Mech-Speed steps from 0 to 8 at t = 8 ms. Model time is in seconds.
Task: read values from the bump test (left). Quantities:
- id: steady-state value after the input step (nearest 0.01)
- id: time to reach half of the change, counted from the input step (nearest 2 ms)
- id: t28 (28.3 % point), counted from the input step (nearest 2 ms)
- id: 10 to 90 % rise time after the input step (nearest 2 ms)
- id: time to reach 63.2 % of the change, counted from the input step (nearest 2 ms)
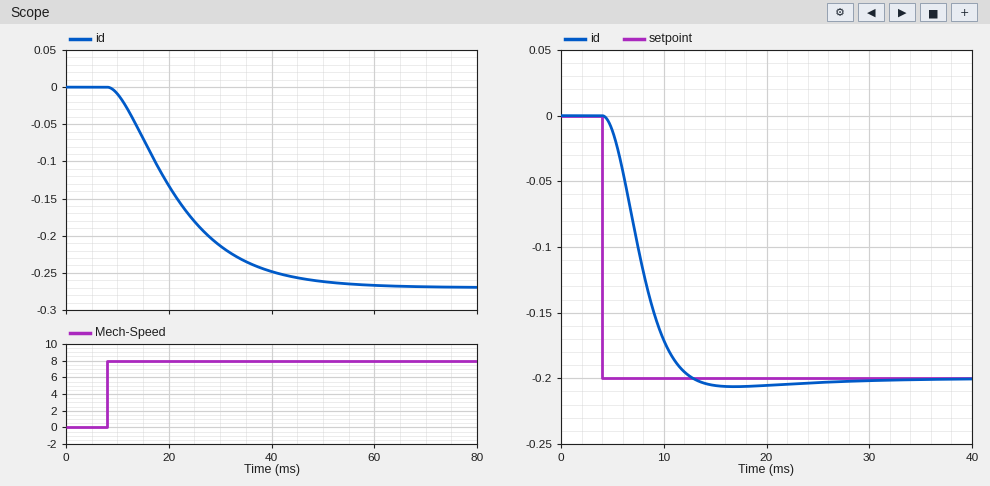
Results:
-0.27
12 ms
8 ms
26 ms
16 ms
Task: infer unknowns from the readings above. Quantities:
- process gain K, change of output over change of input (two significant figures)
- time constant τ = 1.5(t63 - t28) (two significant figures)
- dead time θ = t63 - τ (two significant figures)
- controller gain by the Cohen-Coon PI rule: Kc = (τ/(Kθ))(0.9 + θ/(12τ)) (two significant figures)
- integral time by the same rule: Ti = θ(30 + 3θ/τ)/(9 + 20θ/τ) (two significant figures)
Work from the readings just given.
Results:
-0.034
12 ms
4.0 ms
-82
7.9 ms
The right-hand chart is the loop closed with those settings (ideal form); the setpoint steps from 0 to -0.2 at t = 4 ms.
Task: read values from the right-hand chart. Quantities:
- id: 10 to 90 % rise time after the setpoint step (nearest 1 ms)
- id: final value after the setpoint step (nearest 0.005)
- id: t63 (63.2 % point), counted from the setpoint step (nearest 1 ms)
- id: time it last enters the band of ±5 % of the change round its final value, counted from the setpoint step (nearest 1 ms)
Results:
5 ms
-0.200
4 ms
7 ms
